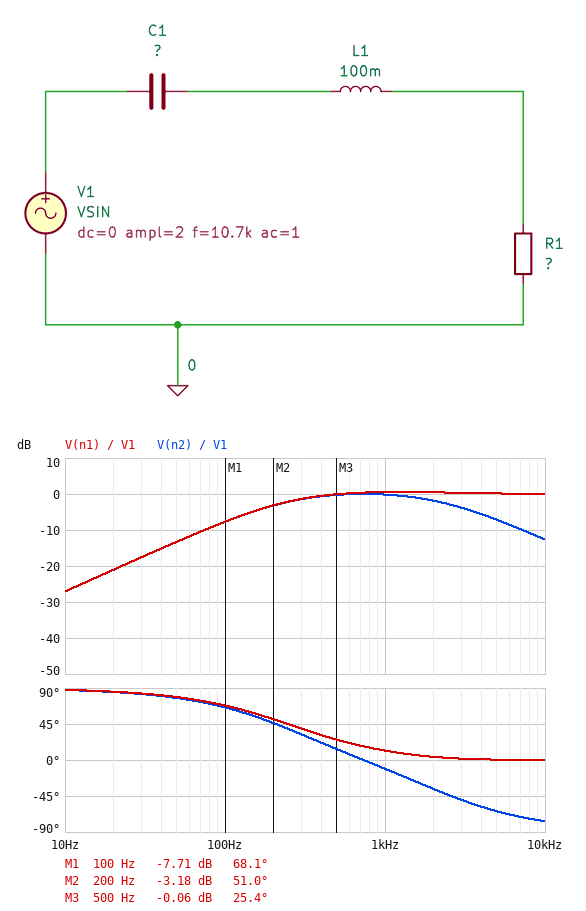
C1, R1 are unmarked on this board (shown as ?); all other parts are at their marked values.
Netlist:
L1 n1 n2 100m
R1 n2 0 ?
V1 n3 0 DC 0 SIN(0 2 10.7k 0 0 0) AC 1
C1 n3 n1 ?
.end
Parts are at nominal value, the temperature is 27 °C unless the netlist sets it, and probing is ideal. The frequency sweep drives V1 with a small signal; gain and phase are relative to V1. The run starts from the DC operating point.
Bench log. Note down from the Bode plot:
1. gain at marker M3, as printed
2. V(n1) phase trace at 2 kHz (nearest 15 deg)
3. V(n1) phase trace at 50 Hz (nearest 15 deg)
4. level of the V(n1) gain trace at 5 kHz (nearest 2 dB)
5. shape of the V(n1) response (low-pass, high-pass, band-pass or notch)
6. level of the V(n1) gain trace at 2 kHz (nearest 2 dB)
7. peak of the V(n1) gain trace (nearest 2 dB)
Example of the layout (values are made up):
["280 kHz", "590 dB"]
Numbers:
["-0.06 dB", "0 deg", "75 deg", "0 dB", "high-pass", "0 dB", "0 dB"]
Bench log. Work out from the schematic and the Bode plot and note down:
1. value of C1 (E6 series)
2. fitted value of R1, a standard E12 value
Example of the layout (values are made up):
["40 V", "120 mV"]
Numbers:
["470 nF", "1.5 kΩ"]
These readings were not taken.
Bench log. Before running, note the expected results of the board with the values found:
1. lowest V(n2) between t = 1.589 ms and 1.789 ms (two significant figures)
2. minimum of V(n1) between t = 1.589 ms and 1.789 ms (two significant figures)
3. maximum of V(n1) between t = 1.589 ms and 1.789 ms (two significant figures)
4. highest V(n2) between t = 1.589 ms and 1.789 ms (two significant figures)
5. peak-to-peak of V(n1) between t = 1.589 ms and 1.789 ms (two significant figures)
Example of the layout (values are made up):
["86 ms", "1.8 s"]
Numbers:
["-440 mV", "-2.0 V", "2.0 V", "430 mV", "4.0 V"]
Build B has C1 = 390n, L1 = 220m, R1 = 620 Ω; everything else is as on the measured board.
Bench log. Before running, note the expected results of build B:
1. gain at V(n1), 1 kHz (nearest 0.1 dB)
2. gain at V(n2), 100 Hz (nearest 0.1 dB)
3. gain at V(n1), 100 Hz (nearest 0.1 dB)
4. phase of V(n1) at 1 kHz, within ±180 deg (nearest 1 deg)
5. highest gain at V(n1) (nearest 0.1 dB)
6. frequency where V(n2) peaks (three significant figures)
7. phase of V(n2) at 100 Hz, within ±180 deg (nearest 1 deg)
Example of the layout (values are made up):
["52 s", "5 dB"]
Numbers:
["2.4 dB", "-16.2 dB", "-16.0 dB", "8 deg", "4.2 dB", "543 Hz", "81 deg"]
